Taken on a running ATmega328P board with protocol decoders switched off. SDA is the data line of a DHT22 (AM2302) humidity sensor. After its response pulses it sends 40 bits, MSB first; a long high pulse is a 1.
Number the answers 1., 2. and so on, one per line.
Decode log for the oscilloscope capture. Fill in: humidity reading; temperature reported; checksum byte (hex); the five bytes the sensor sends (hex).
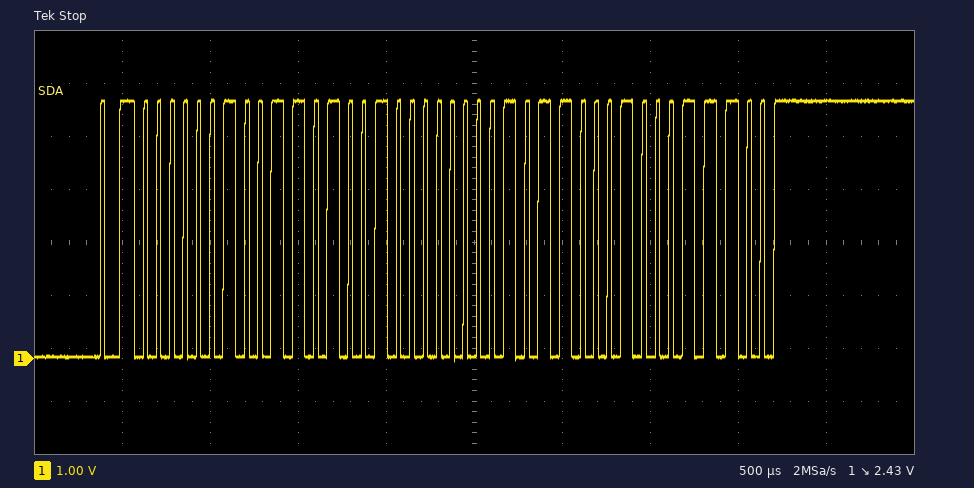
1. 61.7 %
2. 17.7 °C
3. 0x1C
4. 02 69 00 B1 1C
